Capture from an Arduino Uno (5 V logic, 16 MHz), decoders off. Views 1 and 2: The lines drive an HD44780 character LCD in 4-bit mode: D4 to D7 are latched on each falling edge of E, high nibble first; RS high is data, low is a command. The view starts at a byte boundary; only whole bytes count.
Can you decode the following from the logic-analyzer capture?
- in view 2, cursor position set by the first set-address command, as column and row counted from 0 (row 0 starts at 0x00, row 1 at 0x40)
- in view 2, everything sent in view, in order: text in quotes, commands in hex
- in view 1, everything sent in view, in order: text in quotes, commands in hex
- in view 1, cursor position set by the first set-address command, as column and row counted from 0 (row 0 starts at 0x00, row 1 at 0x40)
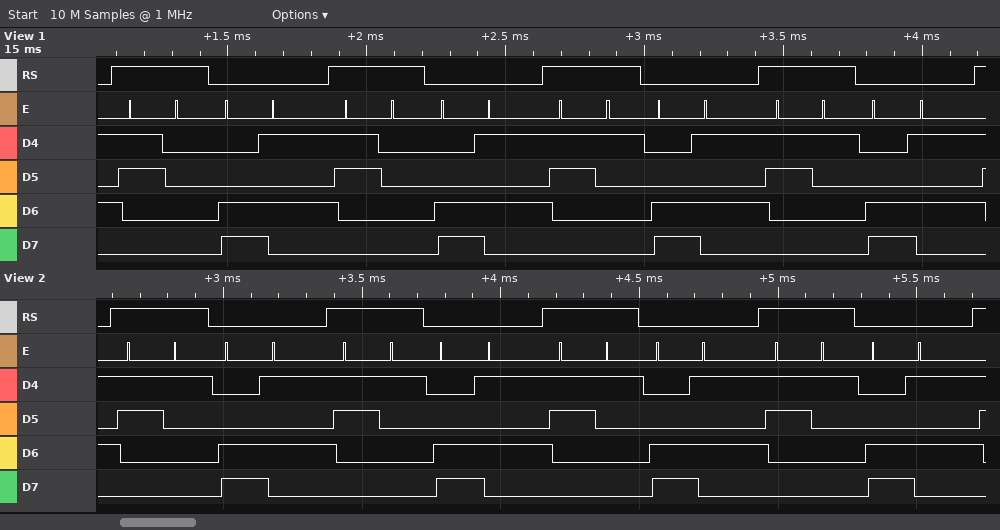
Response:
column 5, row 1
"1" 0xC5 "1" 0xC5 "1" 0xC5 "1" 0xC5
"0" 0xC5 "0" 0xC5 "1" 0xC5 "1" 0xC5
column 5, row 1
